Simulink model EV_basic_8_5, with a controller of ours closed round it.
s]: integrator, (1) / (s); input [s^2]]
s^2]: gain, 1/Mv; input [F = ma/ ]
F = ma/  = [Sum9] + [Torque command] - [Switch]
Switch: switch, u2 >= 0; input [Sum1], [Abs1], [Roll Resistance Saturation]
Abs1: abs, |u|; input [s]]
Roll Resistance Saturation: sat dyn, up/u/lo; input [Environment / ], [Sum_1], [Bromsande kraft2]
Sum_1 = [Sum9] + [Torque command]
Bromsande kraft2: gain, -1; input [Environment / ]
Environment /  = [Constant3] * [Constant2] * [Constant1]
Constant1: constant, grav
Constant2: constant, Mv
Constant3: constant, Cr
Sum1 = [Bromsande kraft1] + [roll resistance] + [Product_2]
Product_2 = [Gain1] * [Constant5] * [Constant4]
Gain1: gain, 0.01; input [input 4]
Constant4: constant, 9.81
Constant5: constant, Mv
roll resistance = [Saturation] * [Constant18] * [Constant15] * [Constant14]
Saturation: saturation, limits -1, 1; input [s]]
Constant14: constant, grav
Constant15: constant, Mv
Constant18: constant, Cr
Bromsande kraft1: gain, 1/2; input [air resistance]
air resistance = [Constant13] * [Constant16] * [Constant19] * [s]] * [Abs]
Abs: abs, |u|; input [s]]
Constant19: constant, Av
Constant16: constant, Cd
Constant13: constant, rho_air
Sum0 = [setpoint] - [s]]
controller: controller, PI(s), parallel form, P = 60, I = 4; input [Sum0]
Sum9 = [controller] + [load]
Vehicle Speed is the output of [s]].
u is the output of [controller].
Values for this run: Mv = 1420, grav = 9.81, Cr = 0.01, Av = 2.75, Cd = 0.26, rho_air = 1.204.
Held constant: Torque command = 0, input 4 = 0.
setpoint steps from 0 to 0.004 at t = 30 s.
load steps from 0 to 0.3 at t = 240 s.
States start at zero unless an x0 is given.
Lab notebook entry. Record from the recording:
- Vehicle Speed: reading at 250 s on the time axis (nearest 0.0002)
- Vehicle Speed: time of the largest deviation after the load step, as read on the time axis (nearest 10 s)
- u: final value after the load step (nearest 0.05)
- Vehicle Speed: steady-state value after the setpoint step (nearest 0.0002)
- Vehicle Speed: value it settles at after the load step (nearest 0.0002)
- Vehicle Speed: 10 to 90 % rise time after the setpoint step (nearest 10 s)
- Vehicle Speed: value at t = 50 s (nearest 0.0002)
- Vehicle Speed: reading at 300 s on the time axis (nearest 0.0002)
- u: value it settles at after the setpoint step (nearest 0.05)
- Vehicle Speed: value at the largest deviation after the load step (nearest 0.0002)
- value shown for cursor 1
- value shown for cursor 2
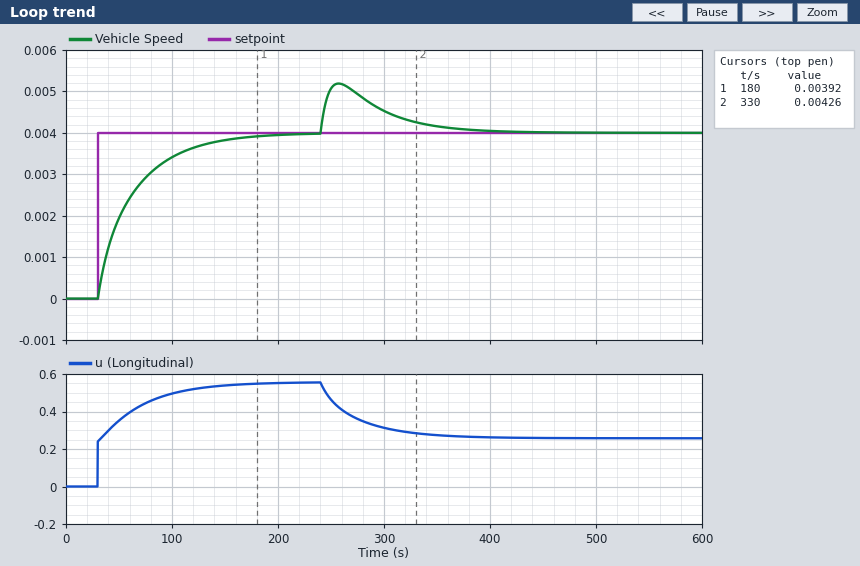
0.0050
260 s
0.25
0.0040
0.0040
80 s
0.0020
0.0046
0.55
0.0052
0.00392
0.00426
